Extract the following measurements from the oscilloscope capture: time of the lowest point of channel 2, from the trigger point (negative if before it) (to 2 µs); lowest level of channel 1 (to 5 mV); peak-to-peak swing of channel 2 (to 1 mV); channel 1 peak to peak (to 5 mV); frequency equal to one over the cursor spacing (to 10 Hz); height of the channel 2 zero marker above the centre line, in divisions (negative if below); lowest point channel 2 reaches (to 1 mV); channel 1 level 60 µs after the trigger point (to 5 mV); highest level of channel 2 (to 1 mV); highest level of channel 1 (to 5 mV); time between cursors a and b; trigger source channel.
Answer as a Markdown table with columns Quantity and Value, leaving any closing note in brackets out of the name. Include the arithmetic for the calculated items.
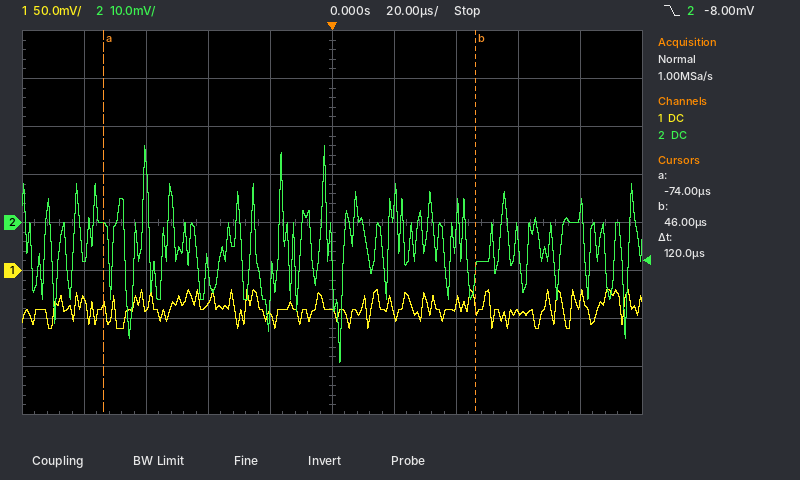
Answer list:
| Quantity | Value |
|---|---|
| time of the lowest point of channel 2, from the trigger point (negative if before it) | +2 µs |
| lowest level of channel 1 | -60 mV |
| peak-to-peak swing of channel 2 | 16 mV − (-29 mV) = 45 mV |
| channel 1 peak to peak | -20 mV − (-60 mV) = 40 mV |
| frequency equal to one over the cursor spacing | 1 / 120 µs ≈ 8.33 kHz |
| height of the channel 2 zero marker above the centre line, in divisions | 0.0 div |
| lowest point channel 2 reaches | -29 mV |
| channel 1 level 60 µs after the trigger point | -45 mV |
| highest level of channel 2 | 16 mV |
| highest level of channel 1 | -20 mV |
| time between cursors a and b | 120 µs |
| trigger source channel | channel 2 |
